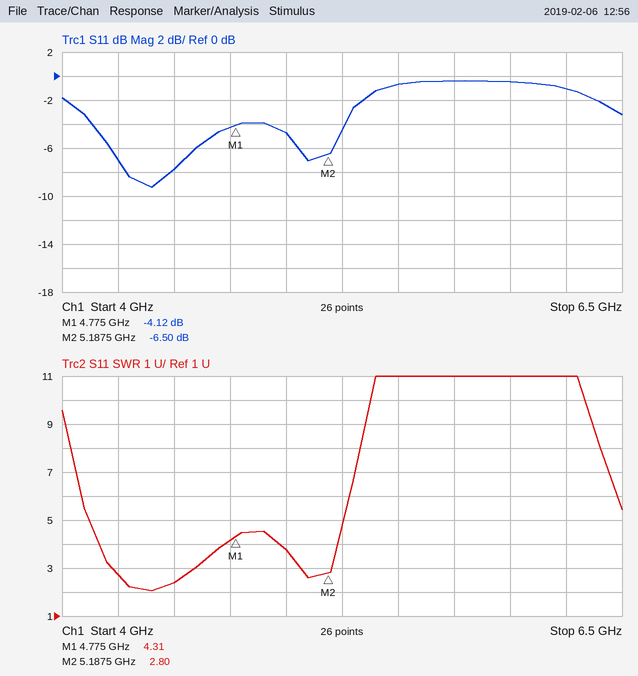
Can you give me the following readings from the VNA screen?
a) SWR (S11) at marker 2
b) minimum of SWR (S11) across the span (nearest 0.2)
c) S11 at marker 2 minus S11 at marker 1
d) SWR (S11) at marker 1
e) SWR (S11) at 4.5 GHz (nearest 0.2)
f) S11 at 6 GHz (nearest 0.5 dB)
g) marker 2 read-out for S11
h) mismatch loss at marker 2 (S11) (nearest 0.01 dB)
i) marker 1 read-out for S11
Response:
2.80
2.0
-2.38 dB
4.31
2.4
-0.5 dB
-6.50 dB
1.10 dB
-4.12 dB
